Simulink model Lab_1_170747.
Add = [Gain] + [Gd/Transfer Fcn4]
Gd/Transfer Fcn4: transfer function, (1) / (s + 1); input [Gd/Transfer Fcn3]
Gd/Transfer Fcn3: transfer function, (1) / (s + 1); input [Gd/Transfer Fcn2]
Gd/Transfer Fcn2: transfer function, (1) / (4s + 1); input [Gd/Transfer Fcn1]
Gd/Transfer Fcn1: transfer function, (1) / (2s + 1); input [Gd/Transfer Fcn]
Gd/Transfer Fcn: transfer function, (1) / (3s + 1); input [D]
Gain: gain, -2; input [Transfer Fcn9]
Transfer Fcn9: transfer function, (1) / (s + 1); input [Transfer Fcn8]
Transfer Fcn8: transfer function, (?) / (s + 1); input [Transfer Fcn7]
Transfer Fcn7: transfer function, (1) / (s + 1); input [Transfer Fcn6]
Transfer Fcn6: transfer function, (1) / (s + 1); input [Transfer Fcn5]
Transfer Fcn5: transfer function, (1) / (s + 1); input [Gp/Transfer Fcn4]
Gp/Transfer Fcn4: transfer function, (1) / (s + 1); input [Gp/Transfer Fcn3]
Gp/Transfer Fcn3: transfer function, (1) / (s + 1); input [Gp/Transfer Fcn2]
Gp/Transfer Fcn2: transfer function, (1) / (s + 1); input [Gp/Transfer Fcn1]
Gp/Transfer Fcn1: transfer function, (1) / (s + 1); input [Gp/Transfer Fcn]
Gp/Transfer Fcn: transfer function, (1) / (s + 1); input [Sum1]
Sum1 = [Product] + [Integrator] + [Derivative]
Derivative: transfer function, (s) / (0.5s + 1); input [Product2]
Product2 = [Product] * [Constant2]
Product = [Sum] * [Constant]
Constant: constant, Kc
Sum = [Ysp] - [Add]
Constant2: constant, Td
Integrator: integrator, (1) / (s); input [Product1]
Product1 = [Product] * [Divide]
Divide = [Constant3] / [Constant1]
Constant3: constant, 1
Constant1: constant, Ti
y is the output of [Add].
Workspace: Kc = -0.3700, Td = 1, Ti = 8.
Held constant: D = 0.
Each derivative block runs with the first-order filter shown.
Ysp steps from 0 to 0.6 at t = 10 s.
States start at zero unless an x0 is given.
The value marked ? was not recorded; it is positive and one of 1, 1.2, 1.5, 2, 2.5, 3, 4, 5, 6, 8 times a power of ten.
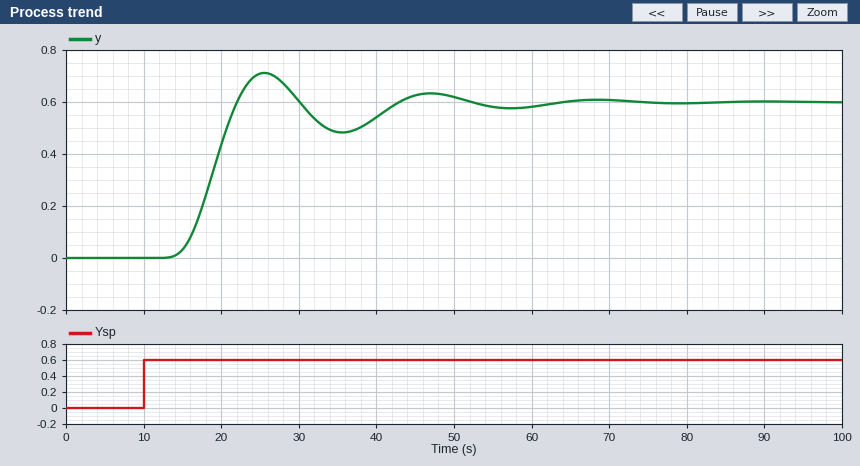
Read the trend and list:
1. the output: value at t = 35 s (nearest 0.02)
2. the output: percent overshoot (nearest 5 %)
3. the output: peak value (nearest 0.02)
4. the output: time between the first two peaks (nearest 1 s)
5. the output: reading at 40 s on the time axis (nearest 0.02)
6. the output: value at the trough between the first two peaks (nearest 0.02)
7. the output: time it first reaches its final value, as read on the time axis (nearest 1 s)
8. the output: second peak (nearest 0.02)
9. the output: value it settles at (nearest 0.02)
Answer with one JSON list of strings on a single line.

["0.48", "20 %", "0.72", "21 s", "0.54", "0.48", "22 s", "0.64", "0.60"]
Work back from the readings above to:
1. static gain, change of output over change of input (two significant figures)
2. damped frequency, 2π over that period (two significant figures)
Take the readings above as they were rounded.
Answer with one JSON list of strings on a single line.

["1.0", "0.30 rad/s"]
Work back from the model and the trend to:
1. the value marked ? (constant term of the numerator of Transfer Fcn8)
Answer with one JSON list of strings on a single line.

["1.2"]
